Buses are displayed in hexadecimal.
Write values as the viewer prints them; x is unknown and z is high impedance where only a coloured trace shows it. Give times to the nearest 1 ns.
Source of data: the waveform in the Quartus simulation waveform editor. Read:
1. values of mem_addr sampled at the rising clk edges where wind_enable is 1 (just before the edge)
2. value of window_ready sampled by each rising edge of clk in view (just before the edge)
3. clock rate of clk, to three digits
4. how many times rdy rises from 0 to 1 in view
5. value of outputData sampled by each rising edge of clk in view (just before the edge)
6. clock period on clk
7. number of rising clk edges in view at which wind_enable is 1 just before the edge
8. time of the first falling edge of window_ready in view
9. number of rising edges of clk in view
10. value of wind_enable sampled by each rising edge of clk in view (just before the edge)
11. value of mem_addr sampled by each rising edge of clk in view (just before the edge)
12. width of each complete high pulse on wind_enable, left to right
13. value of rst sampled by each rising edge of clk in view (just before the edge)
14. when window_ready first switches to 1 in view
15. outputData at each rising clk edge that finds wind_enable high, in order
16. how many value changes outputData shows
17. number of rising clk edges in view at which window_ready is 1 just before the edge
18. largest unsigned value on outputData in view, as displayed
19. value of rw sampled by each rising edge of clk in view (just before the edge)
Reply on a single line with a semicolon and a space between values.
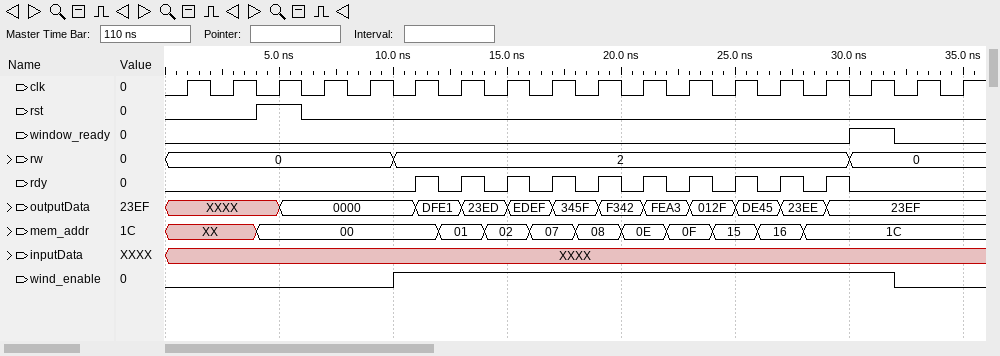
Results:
00, 01, 02, 07, 08, 0E, 0F, 15, 16, 1C, 1C; 0 0 0 0 0 0 0 0 0 0 0 0 0 0 0 1 0 0; 500 MHz; 10; XXXX, XXXX, XXXX, 0000, 0000, 0000, DFE1, 23ED, EDEF, 345F, F342, FEA3, 012F, DE45, 23EE, 23EF, 23EF, 23EF; 2 ns; 11; 32 ns; 18; 0 0 0 0 0 1 1 1 1 1 1 1 1 1 1 1 0 0; XX, XX, 00, 00, 00, 00, 01, 02, 07, 08, 0E, 0F, 15, 16, 1C, 1C, 1C, 1C; 22 ns; 0 0 1 0 0 0 0 0 0 0 0 0 0 0 0 0 0 0; 30 ns; 0000, DFE1, 23ED, EDEF, 345F, F342, FEA3, 012F, DE45, 23EE, 23EF; 11; 1; FEA3; 0, 0, 0, 0, 0, 2, 2, 2, 2, 2, 2, 2, 2, 2, 2, 0, 0, 0
